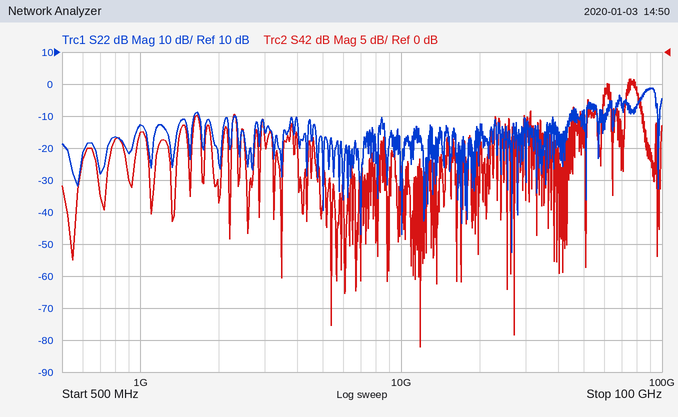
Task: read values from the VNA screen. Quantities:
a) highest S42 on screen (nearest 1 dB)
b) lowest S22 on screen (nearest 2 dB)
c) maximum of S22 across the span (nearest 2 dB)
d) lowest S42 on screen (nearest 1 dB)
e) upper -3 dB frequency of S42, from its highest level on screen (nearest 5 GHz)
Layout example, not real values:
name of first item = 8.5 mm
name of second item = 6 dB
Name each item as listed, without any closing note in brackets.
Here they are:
highest S42 on screen = -4 dB
lowest S22 on screen = -52 dB
maximum of S22 across the span = -2 dB
lowest S42 on screen = -46 dB
upper -3 dB frequency of S42, from its highest level on screen = 80 GHz
